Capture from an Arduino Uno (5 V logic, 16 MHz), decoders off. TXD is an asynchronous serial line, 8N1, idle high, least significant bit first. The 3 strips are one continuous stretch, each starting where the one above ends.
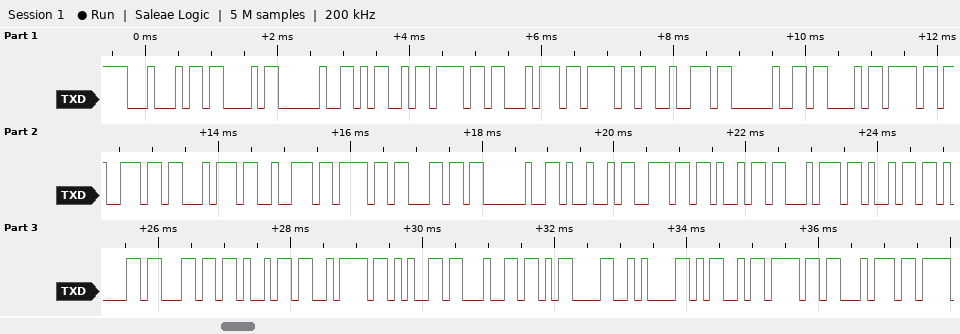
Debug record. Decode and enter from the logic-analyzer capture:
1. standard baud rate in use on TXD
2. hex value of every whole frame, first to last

9600 baud
0x44 0x43 0x20 0x4D 0x6F 0x74 0x6F 0x72 0x20 0x43 0x6F 0x6E 0x74 0x72 0x6F 0x6C 0x20 0x49 0x6E 0x69 0x74 0x69 0x61 0x6C 0x69 0x7A 0x65 0x64 0x0D 0x0A 0x4D 0x6F 0x74
